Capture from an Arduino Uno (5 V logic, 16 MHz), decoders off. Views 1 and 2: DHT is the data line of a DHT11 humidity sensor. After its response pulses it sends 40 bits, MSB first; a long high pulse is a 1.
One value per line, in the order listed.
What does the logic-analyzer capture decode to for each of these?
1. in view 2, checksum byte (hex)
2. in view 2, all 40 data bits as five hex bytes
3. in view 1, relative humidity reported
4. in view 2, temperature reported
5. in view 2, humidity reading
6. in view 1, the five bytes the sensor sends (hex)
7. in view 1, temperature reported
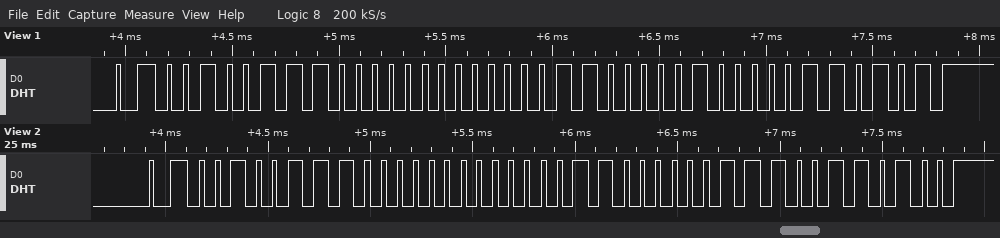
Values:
0x34
27 00 06 07 34
39 %
6.7 °C
39 %
27 00 06 08 35
6.8 °C
